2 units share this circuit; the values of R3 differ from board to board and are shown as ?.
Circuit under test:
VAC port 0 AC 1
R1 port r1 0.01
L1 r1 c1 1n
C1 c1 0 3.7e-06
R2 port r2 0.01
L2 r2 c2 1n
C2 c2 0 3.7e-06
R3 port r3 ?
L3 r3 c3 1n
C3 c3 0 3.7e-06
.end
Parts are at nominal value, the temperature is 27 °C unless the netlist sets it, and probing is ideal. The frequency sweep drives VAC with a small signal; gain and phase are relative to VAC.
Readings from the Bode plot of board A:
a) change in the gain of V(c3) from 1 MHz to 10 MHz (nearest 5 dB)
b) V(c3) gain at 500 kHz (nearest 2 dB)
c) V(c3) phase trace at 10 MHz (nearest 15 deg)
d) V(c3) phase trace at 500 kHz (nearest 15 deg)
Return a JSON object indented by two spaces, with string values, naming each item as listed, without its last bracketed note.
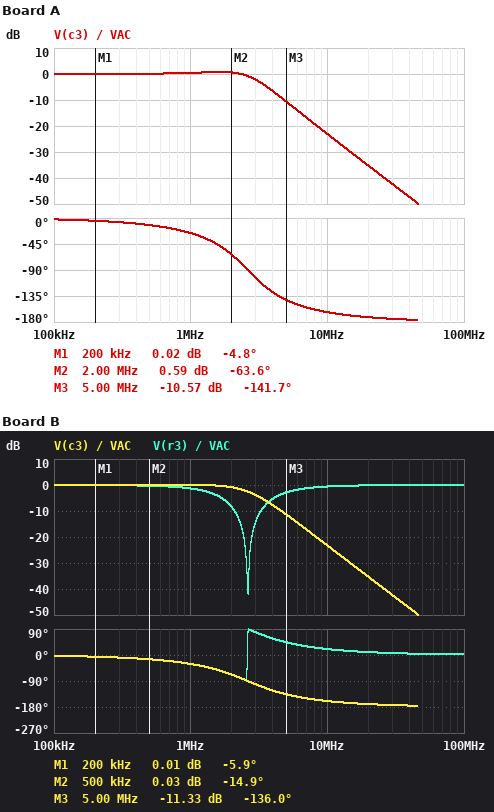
{
  "change in the gain of V(c3) from 1 MHz to 10 MHz": "-25 dB",
  "V(c3) gain at 500 kHz": "0 dB",
  "V(c3) phase trace at 10 MHz": "-165 deg",
  "V(c3) phase trace at 500 kHz": "-15 deg"
}
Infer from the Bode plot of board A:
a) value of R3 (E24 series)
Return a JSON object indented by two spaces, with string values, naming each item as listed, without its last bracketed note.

{
  "value of R3": "0.018 Ω"
}
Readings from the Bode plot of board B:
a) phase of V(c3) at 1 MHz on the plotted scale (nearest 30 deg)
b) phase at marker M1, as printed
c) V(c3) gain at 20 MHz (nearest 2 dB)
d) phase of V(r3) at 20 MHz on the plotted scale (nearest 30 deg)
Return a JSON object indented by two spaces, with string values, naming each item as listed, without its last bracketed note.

{
  "phase of V(c3) at 1 MHz on the plotted scale": "-30 deg",
  "phase at marker M1, as printed": "-5.9 deg",
  "V(c3) gain at 20 MHz": "-36 dB",
  "phase of V(r3) at 20 MHz on the plotted scale": "0 deg"
}
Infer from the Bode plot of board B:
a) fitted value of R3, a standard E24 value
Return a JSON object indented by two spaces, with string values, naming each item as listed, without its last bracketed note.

{
  "fitted value of R3, a standard E24 value": "0.022 Ω"
}
